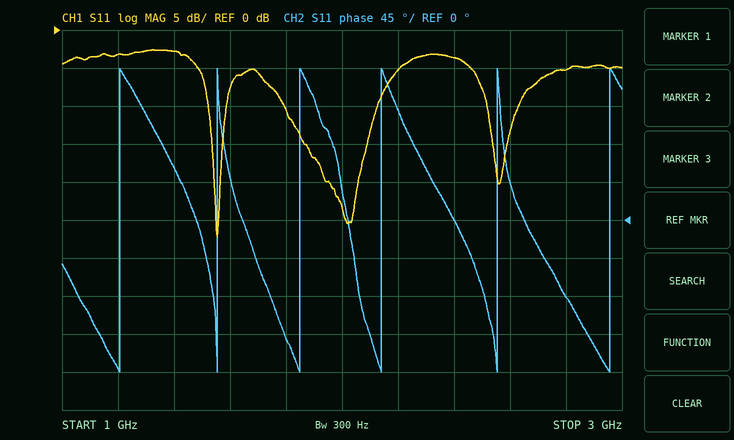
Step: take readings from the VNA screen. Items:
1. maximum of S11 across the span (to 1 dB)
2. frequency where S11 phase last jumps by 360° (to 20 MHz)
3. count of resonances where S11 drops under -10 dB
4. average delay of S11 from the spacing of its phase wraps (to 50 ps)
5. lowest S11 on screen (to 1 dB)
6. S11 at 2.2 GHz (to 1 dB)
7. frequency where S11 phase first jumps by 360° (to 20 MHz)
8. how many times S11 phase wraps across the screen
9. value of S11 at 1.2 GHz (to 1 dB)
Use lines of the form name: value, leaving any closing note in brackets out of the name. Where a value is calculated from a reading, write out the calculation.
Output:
maximum of S11 across the span: -3 dB
frequency where S11 phase last jumps by 360°: 2.96 GHz
count of resonances where S11 drops under -10 dB: 3
average delay of S11 from the spacing of its phase wraps: 5 cycles / (2.96 GHz − 1.20 GHz) ≈ 2.84 ns, so 2.85 ns to the nearest 50 ps
lowest S11 on screen: -27 dB
S11 at 2.2 GHz: -5 dB
frequency where S11 phase first jumps by 360°: 1.20 GHz
how many times S11 phase wraps across the screen: 6
value of S11 at 1.2 GHz: -3 dB
